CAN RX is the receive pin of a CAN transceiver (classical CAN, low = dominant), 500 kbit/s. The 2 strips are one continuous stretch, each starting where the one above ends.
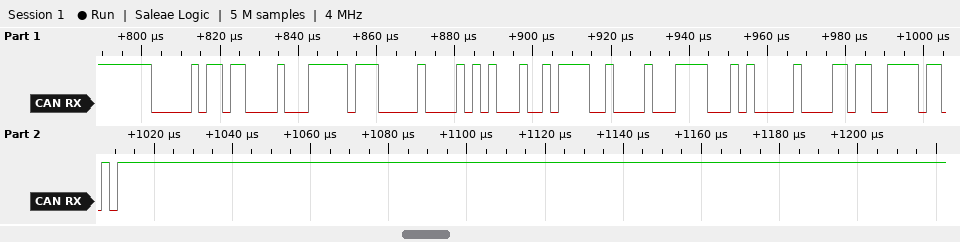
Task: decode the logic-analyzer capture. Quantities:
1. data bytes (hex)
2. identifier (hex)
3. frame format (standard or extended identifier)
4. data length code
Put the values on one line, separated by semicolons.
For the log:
FF 00 54 4B C8 47 8A 00; 0x036; standard; 8
